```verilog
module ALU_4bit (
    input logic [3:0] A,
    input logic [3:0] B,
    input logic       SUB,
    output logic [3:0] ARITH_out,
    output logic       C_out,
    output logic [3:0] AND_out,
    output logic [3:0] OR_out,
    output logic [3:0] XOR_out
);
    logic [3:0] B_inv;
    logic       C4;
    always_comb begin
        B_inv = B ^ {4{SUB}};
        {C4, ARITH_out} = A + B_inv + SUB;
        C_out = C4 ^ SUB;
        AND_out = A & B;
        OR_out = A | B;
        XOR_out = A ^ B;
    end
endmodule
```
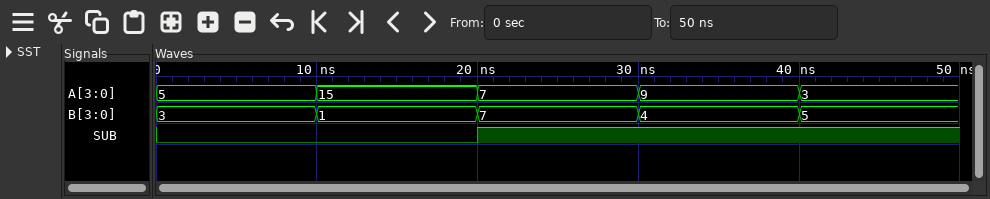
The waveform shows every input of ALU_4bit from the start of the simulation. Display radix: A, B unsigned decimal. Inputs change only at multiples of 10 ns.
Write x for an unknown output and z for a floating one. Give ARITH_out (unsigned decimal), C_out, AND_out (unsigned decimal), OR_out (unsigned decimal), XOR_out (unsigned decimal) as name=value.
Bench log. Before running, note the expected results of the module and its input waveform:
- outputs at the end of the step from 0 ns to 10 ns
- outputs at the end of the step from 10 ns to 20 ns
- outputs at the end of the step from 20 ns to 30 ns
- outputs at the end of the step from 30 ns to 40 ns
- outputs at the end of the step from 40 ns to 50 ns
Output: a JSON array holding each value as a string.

["ARITH_out=8, C_out=0, AND_out=1, OR_out=7, XOR_out=6", "ARITH_out=0, C_out=1, AND_out=1, OR_out=15, XOR_out=14", "ARITH_out=0, C_out=0, AND_out=7, OR_out=7, XOR_out=0", "ARITH_out=5, C_out=0, AND_out=0, OR_out=13, XOR_out=13", "ARITH_out=14, C_out=1, AND_out=1, OR_out=7, XOR_out=6"]
